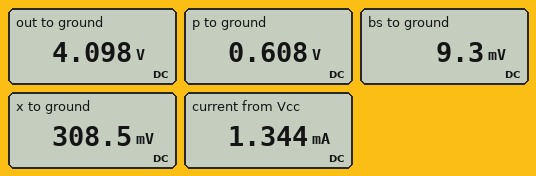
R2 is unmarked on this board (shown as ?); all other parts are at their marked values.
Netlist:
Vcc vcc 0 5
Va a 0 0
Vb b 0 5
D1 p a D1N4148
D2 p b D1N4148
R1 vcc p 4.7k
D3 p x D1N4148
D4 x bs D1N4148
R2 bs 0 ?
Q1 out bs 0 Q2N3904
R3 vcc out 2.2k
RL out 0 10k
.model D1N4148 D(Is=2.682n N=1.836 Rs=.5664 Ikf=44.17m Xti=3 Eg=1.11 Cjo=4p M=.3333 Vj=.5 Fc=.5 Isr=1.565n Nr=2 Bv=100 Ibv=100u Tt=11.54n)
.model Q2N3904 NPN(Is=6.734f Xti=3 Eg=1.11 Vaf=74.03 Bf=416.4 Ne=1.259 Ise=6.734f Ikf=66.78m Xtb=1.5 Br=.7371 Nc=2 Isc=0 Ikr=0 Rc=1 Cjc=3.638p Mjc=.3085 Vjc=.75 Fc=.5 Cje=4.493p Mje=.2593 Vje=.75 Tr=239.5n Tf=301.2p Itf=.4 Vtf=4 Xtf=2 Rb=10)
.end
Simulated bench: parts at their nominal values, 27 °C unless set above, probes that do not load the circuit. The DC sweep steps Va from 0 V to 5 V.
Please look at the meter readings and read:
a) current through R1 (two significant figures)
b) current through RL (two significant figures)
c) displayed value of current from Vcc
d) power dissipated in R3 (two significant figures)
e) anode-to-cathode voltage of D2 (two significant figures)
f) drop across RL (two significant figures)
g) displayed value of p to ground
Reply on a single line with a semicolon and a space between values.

930 µA; 410 µA; 1.344 mA; 370 µW; -4.4 V; 4.1 V; 0.608 V
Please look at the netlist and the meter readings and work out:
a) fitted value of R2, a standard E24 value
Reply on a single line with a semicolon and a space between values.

5.1 kΩ
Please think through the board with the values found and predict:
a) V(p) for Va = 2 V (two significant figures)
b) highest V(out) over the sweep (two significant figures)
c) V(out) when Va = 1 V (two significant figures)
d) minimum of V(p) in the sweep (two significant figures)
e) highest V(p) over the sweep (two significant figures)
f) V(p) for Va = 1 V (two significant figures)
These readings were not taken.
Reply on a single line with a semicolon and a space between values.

1.9 V; 4.1 V; 4.0 V; 610 mV; 1.9 V; 1.6 V
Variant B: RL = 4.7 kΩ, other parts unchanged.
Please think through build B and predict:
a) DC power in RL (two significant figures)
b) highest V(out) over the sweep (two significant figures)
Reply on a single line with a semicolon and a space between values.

2.5 mW; 3.4 V
